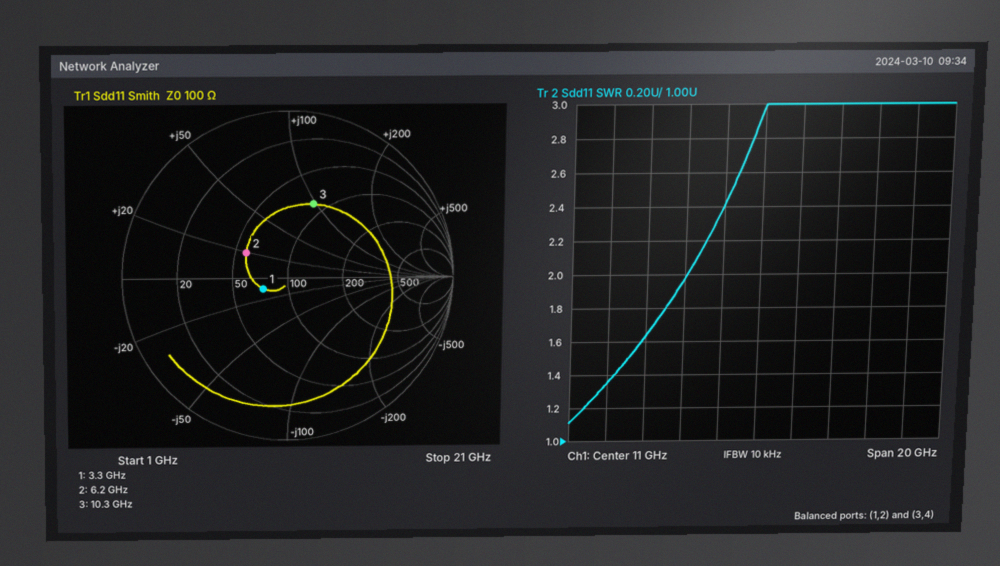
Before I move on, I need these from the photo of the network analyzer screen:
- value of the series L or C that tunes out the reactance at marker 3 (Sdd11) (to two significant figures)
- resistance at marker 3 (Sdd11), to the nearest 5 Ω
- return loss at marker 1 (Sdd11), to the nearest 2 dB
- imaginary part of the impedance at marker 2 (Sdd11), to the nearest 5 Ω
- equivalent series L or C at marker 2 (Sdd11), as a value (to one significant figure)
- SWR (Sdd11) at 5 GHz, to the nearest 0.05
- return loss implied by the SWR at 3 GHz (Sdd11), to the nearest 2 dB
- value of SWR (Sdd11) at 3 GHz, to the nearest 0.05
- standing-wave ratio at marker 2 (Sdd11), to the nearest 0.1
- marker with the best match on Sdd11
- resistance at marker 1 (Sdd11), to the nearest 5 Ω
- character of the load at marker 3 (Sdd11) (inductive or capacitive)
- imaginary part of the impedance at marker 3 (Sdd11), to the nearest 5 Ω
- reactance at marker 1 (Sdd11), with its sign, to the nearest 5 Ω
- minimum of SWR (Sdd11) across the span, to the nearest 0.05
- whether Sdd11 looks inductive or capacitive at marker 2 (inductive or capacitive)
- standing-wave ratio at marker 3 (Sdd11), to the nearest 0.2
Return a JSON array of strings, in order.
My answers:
["160 fF", "85 Ω", "16 dB", "+20 Ω", "500 pH", "1.65", "16 dB", "1.35", "1.8", "marker 1", "75 Ω", "inductive", "+95 Ω", "-10 Ω", "1.10", "inductive", "2.8"]
